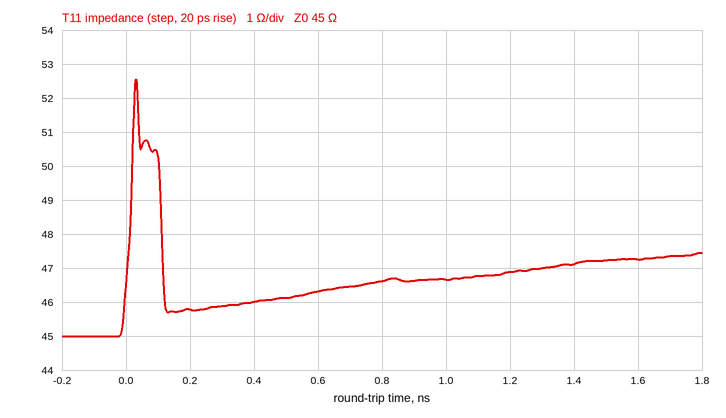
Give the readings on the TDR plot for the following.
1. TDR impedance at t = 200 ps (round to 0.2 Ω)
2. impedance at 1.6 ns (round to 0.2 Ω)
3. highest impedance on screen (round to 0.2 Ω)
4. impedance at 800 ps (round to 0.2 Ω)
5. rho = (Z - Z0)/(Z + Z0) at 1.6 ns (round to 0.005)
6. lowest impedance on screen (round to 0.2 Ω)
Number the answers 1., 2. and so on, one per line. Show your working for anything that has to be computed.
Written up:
1. 45.8 Ω
2. 47.2 Ω
3. 52.6 Ω
4. 46.6 Ω
5. (47.2 − 45)/(47.2 + 45) ≈ +0.0239, so +0.025 to the nearest 0.005
6. 45.0 Ω
